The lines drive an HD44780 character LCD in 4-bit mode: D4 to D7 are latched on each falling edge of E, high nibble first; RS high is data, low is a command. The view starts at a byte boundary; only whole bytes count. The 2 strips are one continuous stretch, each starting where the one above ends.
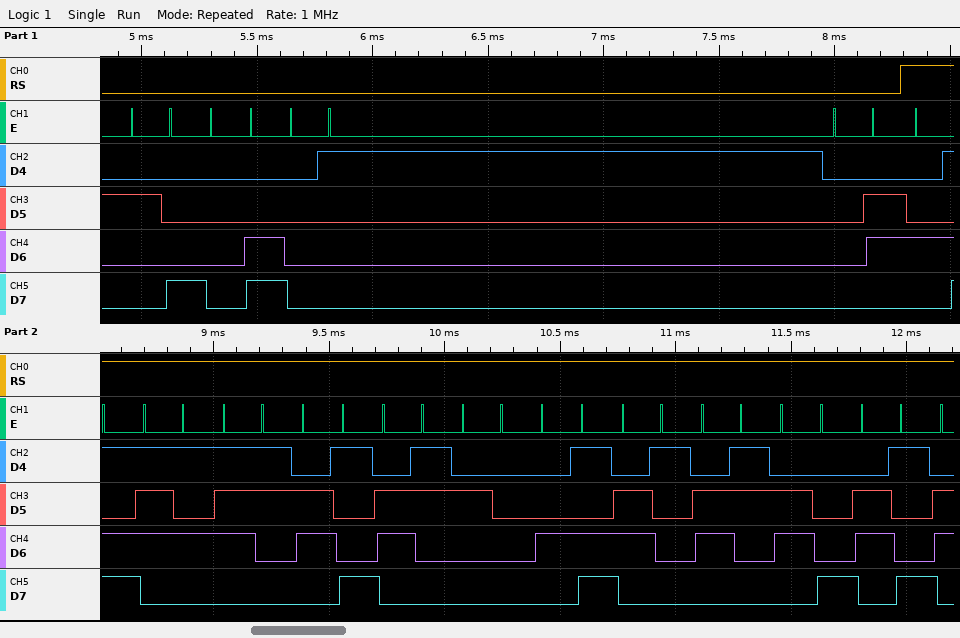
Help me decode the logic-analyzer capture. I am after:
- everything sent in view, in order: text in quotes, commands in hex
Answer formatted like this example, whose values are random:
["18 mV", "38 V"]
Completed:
["0x28 0x0C 0x01 0x06 \"Music Machi\""]
